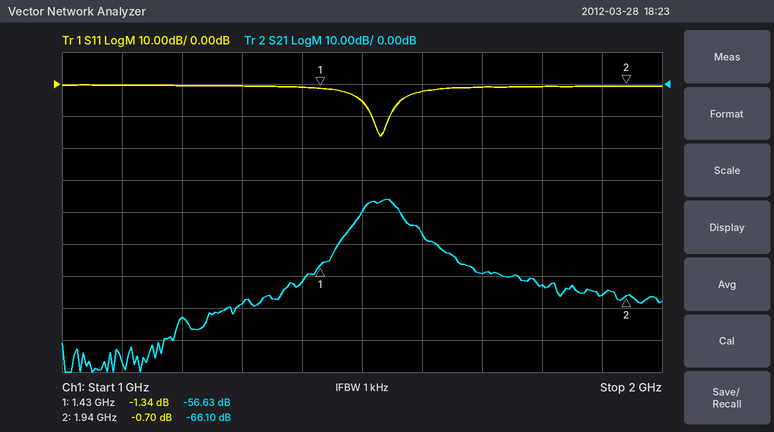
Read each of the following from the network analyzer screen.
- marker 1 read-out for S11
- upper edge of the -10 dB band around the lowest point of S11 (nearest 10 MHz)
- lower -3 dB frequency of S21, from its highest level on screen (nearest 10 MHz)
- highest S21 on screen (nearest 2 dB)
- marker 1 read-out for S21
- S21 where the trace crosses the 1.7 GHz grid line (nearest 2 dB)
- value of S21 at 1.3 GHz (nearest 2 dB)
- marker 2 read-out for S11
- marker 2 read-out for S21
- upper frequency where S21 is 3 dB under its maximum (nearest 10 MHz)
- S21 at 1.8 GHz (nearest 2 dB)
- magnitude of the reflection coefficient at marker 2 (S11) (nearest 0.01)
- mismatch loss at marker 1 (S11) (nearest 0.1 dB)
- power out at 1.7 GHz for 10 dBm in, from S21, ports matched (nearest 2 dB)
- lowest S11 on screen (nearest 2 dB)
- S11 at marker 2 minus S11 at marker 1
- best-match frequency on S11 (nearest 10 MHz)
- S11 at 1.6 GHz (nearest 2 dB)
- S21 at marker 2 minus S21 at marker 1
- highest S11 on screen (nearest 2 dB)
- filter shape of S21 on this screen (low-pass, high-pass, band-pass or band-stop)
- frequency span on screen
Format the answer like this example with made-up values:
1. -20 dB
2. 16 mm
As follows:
1. -1.34 dB
2. 1.55 GHz
3. 1.50 GHz
4. -36 dB
5. -56.63 dB
6. -60 dB
7. -68 dB
8. -0.70 dB
9. -66.10 dB
10. 1.56 GHz
11. -62 dB
12. 0.92
13. 5.8 dB
14. -50 dBm
15. -16 dB
16. 0.64 dB
17. 1.53 GHz
18. -2 dB
19. -9.47 dB
20. 0 dB
21. band-pass
22. 1 GHz
